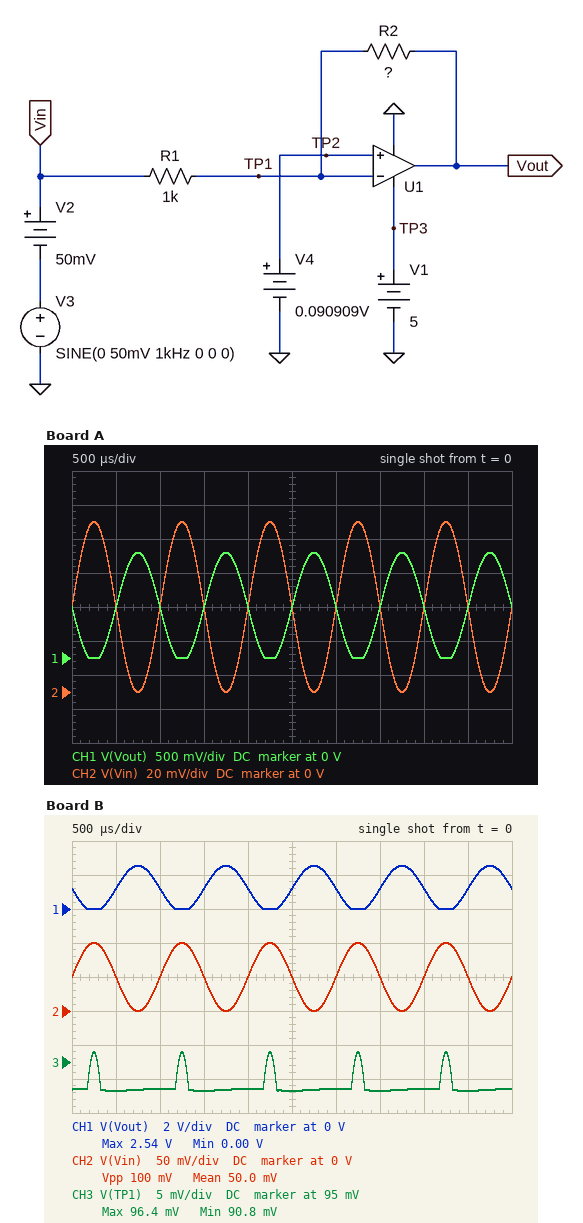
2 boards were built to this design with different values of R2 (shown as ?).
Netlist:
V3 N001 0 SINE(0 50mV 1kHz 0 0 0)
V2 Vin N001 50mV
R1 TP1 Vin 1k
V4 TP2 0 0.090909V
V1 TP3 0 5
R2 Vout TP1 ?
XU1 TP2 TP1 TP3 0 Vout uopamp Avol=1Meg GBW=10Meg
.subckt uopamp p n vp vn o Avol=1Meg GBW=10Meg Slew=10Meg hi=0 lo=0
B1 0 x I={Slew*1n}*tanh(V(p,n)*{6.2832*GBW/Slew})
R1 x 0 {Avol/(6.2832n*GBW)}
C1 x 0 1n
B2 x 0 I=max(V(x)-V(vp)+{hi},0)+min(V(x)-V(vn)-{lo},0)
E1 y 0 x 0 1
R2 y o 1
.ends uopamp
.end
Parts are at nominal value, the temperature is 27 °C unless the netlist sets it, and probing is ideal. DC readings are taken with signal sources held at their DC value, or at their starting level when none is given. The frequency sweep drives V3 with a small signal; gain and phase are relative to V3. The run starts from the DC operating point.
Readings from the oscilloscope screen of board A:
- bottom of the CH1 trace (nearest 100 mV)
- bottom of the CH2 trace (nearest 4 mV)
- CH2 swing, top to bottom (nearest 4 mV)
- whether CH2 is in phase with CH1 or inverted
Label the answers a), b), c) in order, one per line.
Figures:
a) 0 V
b) 0 V
c) 100 mV
d) inverted
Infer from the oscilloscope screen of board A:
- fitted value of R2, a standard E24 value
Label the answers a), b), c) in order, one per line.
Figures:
a) 16 kΩ
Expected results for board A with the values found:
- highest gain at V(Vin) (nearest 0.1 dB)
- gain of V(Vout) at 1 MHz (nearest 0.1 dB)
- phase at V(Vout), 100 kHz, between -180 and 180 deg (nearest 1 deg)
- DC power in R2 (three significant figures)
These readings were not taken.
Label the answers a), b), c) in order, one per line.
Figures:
a) 0 dB
b) 18.2 dB
c) 170 deg
d) 26.8 µW
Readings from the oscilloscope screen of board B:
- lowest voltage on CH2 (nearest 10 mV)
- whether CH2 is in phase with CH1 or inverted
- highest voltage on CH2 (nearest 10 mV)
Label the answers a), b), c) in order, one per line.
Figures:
a) 0 V
b) inverted
c) 100 mV
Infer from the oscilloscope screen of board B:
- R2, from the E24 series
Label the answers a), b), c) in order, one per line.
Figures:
a) 27 kΩ
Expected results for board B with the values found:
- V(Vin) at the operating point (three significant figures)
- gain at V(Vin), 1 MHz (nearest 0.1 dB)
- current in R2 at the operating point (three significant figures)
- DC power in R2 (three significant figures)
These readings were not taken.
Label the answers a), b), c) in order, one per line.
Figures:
a) 50.0 mV
b) 0 dB
c) 40.9 µA
d) 45.2 µW
